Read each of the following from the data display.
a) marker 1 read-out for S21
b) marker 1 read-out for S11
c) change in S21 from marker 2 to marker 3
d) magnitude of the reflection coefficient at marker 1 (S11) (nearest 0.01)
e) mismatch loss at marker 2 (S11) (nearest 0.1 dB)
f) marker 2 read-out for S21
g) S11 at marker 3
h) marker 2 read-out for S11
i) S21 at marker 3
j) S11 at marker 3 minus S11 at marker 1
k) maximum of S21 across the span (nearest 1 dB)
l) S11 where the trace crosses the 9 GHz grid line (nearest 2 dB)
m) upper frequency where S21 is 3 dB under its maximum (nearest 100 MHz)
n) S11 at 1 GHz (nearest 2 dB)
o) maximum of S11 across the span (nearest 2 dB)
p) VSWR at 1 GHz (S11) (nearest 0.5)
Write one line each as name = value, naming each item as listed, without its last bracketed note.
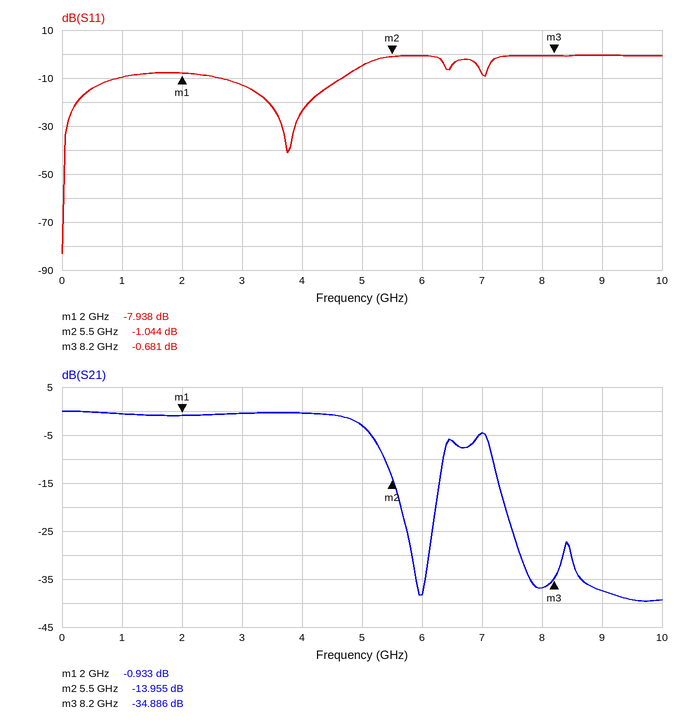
marker 1 read-out for S21 = -0.933 dB
marker 1 read-out for S11 = -7.938 dB
change in S21 from marker 2 to marker 3 = -20.931 dB
magnitude of the reflection coefficient at marker 1 (S11) = 0.40
mismatch loss at marker 2 (S11) = 6.7 dB
marker 2 read-out for S21 = -13.955 dB
S11 at marker 3 = -0.681 dB
marker 2 read-out for S11 = -1.044 dB
S21 at marker 3 = -34.886 dB
S11 at marker 3 minus S11 at marker 1 = 7.257 dB
maximum of S21 across the span = 0 dB
S11 where the trace crosses the 9 GHz grid line = 0 dB
upper frequency where S21 is 3 dB under its maximum = 5.0 GHz
S11 at 1 GHz = -10 dB
maximum of S11 across the span = 0 dB
VSWR at 1 GHz (S11) = 2.0
